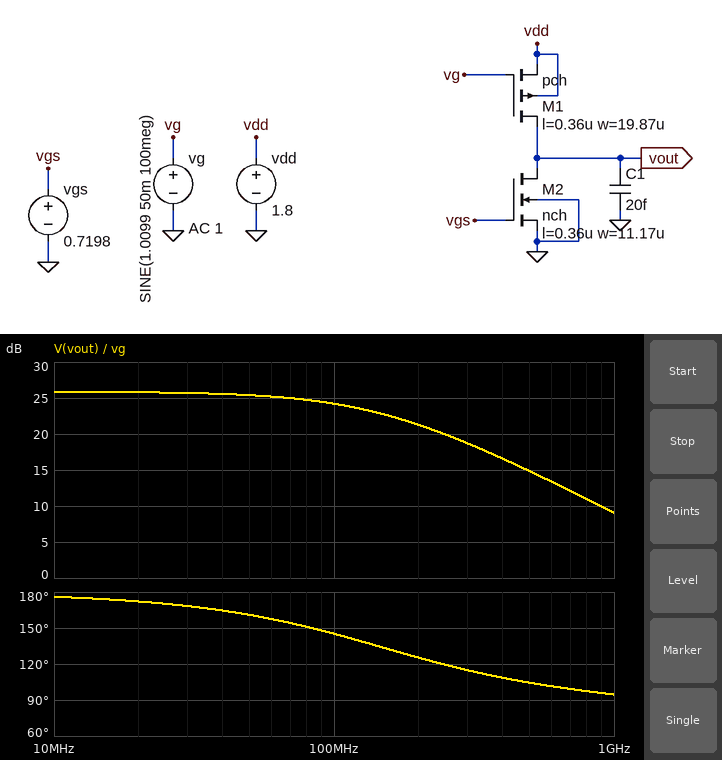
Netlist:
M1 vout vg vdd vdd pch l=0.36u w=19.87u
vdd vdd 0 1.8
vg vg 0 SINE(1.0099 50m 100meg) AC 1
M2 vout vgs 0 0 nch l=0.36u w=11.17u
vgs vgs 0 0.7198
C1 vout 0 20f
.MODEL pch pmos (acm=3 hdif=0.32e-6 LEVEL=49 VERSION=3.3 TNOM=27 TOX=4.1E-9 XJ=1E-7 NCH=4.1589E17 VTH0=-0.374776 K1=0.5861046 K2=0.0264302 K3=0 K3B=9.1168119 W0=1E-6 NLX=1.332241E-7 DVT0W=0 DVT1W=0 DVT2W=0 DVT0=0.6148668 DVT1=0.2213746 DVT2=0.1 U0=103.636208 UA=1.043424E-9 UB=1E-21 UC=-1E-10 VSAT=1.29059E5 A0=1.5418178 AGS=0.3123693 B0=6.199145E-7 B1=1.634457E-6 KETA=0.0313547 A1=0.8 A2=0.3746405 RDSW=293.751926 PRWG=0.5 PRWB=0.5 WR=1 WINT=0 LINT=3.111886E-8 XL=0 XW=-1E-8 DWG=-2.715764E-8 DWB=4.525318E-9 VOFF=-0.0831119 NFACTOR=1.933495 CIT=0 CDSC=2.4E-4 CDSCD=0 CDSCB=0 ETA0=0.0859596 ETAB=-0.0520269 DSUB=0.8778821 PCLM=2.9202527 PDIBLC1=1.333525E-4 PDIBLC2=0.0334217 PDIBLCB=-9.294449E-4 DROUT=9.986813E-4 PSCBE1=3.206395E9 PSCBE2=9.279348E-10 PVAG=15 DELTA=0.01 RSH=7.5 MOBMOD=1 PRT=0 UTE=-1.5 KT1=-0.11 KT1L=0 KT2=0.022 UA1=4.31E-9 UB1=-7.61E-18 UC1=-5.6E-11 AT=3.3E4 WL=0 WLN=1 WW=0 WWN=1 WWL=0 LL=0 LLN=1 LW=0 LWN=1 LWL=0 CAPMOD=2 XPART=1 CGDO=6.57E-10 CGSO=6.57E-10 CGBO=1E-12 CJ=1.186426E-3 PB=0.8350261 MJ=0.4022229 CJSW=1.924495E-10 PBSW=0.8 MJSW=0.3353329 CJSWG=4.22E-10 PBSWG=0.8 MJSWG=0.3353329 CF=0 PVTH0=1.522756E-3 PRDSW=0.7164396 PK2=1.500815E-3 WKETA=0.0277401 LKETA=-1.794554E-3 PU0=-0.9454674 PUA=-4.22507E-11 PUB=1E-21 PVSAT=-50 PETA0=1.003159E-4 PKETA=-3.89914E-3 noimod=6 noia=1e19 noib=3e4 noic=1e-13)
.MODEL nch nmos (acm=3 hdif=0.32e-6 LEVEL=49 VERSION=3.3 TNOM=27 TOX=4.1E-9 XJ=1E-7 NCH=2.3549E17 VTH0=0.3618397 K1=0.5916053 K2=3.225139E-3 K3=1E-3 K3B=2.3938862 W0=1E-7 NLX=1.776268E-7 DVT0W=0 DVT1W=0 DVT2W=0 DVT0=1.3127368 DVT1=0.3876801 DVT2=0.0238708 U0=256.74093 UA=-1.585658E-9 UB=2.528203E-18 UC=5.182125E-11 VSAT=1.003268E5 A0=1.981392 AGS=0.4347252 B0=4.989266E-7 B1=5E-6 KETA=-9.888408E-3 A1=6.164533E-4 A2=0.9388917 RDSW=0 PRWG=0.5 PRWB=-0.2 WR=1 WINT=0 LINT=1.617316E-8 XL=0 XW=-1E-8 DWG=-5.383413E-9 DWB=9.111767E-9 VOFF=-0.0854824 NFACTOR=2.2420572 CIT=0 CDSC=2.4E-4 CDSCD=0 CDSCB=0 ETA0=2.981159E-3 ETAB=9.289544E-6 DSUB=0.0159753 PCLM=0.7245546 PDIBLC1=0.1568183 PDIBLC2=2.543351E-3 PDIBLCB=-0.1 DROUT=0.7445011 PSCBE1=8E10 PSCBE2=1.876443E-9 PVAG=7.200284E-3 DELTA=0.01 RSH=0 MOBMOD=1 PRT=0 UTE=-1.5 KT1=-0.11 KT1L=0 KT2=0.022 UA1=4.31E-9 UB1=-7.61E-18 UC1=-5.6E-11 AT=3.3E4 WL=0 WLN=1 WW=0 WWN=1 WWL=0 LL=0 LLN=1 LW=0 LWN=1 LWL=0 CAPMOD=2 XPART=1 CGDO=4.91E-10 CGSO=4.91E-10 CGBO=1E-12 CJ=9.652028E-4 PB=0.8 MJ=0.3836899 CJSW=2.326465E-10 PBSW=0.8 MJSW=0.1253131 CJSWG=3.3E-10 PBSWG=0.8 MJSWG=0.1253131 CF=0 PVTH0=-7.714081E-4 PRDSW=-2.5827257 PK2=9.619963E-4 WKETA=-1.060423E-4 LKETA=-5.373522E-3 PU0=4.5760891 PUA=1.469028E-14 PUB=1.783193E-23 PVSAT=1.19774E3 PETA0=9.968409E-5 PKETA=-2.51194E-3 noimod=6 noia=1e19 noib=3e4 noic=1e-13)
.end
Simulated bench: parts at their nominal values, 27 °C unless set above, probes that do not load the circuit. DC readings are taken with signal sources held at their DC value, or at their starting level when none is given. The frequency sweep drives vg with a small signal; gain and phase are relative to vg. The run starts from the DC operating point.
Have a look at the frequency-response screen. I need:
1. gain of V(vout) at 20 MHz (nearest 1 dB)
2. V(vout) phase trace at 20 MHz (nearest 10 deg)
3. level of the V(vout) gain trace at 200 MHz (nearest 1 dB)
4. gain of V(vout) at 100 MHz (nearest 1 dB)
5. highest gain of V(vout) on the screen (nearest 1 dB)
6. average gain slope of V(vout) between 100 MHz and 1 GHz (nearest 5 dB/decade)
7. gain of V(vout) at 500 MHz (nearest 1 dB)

26 dB
170 deg
21 dB
24 dB
26 dB
-15 dB/decade
15 dB
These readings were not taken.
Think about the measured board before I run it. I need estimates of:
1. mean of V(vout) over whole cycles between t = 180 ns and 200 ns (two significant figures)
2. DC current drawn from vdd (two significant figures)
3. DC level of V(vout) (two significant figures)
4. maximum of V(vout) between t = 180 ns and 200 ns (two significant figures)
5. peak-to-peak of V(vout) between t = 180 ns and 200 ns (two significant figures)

620 mV
240 µA
410 mV
1.3 V
1.2 V
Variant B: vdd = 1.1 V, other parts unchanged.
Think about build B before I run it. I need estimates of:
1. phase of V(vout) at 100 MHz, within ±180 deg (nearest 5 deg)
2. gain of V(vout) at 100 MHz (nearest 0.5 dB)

90 deg
-49.0 dB
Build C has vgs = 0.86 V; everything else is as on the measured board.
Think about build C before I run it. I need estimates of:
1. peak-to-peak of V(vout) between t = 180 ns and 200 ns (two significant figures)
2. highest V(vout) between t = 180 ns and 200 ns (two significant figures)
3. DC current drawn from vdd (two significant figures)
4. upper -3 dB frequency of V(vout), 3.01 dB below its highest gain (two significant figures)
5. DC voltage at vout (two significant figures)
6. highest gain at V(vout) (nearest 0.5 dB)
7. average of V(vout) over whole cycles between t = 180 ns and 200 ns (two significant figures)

51 mV
110 mV
250 µA
4.3 GHz
80 mV
-6.0 dB
82 mV
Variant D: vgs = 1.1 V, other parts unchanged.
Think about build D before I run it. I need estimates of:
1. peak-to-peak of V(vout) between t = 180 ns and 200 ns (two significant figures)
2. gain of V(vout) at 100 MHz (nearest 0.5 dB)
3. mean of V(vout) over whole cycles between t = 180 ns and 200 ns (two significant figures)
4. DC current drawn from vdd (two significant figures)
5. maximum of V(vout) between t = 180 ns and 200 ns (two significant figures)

25 mV
-12.0 dB
45 mV
250 µA
58 mV
